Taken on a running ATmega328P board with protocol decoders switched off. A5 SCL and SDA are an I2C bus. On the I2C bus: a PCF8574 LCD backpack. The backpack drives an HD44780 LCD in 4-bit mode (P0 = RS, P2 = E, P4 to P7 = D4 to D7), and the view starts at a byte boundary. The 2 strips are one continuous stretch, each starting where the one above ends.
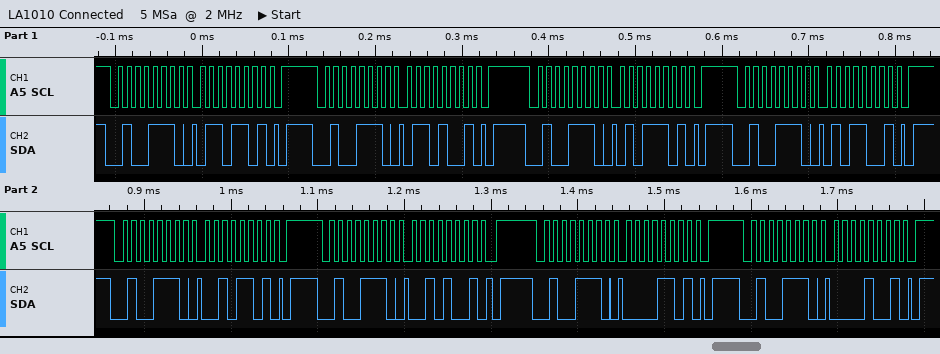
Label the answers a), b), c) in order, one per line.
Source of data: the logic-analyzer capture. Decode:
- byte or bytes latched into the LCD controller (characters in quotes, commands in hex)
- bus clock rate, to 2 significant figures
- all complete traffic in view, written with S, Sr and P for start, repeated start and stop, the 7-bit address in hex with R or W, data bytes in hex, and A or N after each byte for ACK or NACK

a) 'e' ' '
b) 100 kHz
c) S 27W A 6D A P S 27W A 69 A P S 27W A 5D A P S 27W A 59 A P S 27W A 2D A P S 27W A 29 A P S 27W A 0D A P S 27W A 09 A P
